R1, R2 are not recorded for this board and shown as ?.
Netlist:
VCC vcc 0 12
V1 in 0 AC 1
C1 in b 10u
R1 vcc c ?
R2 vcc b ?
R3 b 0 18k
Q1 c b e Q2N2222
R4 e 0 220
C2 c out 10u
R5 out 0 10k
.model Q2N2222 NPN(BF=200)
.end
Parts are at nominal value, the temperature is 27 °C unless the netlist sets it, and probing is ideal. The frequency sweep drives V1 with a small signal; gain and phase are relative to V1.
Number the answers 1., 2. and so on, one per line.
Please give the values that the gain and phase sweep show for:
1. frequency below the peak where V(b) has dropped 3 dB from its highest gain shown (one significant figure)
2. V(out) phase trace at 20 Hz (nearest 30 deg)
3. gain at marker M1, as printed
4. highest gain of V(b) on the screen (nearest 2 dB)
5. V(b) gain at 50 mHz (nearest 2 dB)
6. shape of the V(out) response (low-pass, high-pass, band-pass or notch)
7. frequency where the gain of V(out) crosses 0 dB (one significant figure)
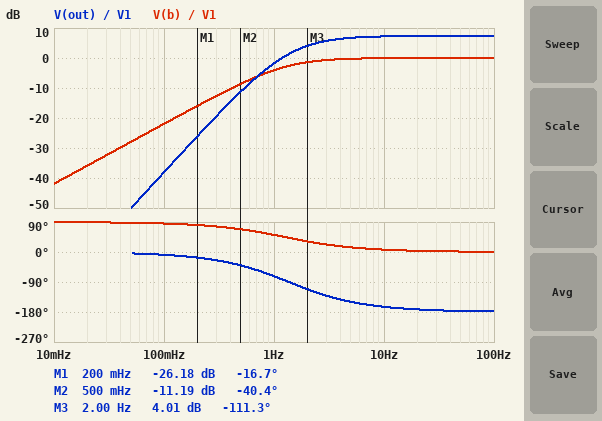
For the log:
1. 1 Hz
2. -180 deg
3. -26.18 dB
4. 0 dB
5. -28 dB
6. high-pass
7. 1 Hz
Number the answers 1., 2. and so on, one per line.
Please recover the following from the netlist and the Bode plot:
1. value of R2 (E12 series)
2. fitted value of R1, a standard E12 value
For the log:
1. 220 kΩ
2. 680 Ω
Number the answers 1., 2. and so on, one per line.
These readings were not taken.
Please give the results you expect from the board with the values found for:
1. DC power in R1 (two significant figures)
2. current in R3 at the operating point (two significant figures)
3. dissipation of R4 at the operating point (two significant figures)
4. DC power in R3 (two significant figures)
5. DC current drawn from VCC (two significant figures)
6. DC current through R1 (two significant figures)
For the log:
1. 170 µW
2. 48 µA
3. 55 µW
4. 42 µW
5. 550 µA
6. 500 µA
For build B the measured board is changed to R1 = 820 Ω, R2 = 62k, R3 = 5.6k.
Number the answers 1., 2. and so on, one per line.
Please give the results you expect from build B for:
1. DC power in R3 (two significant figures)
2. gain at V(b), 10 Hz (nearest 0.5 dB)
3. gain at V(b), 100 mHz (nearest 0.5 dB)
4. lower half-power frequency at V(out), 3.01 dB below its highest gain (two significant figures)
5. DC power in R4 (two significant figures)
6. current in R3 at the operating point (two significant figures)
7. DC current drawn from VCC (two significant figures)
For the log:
1. 170 µW
2. -0.5 dB
3. -30.5 dB
4. 3.9 Hz
5. 180 µW
6. 170 µA
7. 1.1 mA
